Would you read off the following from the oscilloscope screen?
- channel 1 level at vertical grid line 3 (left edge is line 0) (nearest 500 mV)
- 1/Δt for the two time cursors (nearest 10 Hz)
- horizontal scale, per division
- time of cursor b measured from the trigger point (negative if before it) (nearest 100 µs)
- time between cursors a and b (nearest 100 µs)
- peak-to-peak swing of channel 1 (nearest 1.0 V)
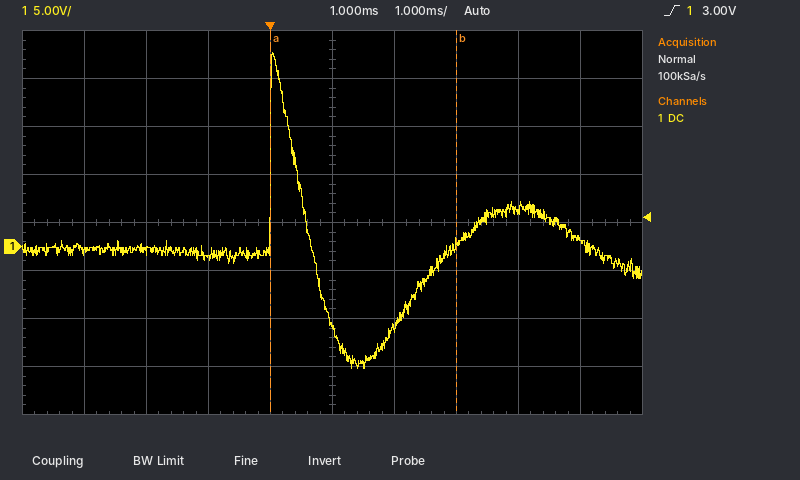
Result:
-1.0 V
330 Hz
1 ms
+3.0 ms
3.0 ms
33.0 V
